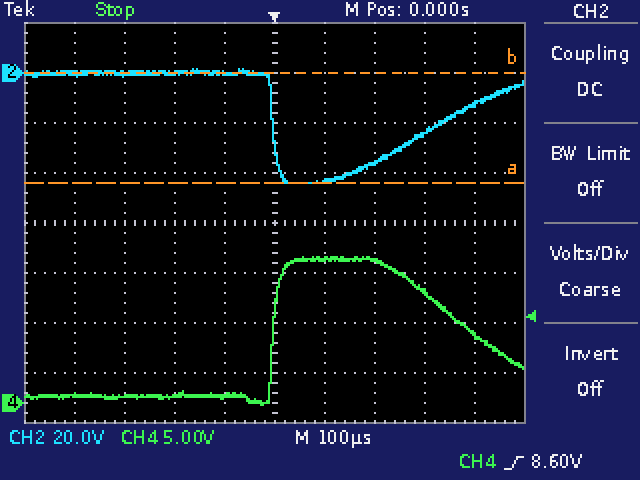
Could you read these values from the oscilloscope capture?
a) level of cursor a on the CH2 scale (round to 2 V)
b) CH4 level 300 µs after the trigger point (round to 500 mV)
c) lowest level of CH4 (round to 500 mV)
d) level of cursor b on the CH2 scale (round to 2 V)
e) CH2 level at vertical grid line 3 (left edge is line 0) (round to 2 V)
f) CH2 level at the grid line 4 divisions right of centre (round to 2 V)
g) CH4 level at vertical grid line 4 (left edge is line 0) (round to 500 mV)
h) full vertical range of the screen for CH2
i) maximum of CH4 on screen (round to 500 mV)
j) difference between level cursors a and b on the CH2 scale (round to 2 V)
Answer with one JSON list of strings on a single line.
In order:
["-44 V", "11.0 V", "0.0 V", "0 V", "0 V", "-12 V", "500 mV", "160 V", "14.5 V", "44 V"]
